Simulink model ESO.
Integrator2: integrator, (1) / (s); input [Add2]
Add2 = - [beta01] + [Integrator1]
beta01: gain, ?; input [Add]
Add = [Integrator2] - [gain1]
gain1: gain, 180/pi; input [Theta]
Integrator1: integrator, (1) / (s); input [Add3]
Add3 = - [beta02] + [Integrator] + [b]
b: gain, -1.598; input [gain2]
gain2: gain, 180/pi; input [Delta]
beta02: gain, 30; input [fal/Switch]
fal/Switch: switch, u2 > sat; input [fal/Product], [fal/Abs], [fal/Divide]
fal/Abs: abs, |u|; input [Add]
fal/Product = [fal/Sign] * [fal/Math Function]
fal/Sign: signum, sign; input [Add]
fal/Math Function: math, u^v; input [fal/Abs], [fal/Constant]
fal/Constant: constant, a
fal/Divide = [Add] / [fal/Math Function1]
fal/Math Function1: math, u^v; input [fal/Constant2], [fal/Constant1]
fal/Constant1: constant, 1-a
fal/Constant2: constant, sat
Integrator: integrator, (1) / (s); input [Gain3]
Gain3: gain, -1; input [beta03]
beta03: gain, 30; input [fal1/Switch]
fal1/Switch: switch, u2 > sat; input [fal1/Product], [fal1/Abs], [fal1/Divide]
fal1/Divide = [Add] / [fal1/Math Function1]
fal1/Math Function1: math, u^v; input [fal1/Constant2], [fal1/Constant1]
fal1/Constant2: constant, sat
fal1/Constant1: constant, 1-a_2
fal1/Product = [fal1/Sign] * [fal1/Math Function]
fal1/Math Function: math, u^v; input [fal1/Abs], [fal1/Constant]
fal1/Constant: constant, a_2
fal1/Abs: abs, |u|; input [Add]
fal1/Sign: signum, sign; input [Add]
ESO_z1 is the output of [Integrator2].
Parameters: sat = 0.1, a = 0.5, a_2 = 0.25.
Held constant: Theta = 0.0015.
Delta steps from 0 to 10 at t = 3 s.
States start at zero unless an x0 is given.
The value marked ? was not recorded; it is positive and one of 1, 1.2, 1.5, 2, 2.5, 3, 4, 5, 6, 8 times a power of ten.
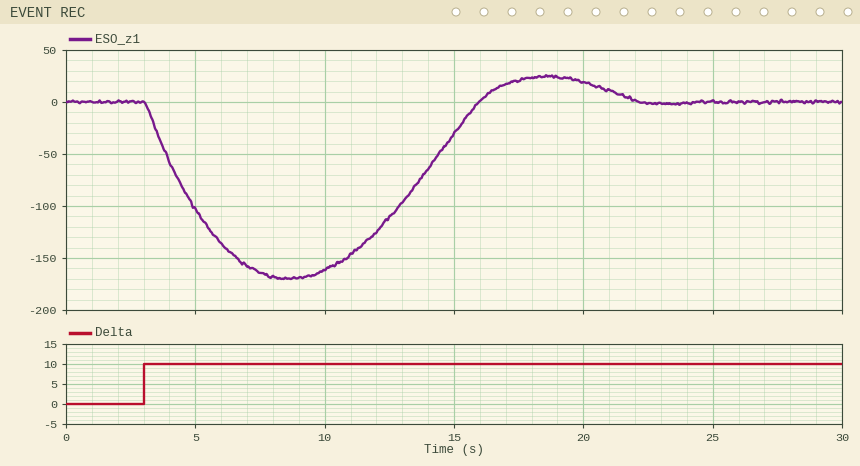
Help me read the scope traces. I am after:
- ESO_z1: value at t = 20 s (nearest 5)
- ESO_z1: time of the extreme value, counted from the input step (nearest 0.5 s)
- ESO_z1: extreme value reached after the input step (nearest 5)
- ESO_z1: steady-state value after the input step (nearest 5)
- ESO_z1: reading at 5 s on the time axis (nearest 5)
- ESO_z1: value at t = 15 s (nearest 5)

20
5.5 s
-170
0
-105
-30
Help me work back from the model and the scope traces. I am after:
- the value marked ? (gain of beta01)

12
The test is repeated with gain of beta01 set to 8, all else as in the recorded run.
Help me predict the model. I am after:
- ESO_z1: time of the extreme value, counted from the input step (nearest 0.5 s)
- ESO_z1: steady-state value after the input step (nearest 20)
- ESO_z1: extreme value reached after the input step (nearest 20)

5.0 s
0
-220
